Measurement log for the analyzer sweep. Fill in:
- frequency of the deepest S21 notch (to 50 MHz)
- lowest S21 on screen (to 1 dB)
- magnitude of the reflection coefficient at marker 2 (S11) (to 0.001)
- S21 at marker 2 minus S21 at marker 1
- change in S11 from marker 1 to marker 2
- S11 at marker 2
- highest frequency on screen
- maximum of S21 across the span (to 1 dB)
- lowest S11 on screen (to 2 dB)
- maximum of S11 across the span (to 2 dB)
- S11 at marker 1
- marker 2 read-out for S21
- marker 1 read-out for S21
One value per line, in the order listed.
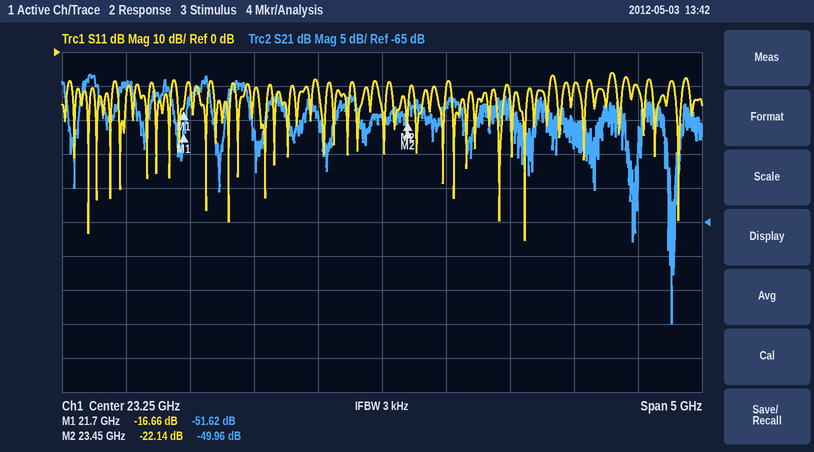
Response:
25.50 GHz
-80 dB
0.078
1.66 dB
-5.48 dB
-22.14 dB
25.75 GHz
-43 dB
-56 dB
-6 dB
-16.66 dB
-49.96 dB
-51.62 dB
